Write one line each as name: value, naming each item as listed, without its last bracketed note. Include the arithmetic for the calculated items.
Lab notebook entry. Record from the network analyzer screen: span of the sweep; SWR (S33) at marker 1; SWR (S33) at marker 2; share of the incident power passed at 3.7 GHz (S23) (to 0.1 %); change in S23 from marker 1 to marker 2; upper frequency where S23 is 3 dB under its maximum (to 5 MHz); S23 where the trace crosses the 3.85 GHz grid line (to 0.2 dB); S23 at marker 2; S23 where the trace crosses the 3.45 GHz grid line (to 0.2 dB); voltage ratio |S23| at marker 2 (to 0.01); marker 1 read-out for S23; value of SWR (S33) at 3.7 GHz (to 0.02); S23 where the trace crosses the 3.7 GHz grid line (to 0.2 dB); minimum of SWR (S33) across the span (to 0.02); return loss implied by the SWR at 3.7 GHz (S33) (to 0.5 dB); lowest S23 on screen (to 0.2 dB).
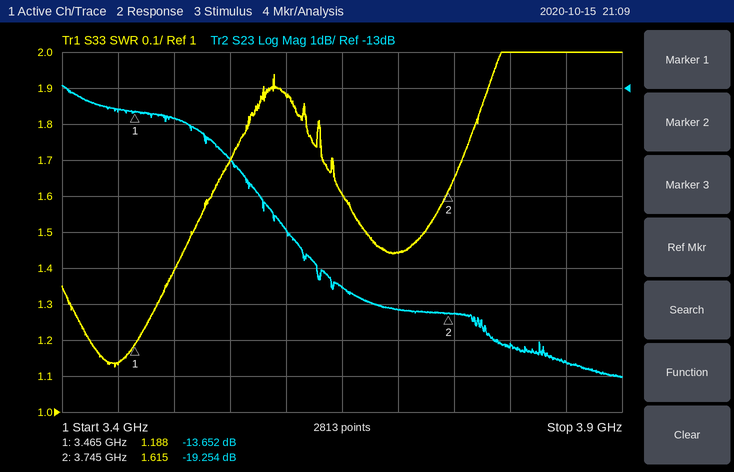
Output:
span of the sweep: 500 MHz
SWR (S33) at marker 1: 1.188
SWR (S33) at marker 2: 1.615
share of the incident power passed at 3.7 GHz (S23): 10^(-19.2/10) ≈ 1.2 %
change in S23 from marker 1 to marker 2: -19.254 − (-13.652) = -5.602 dB
upper frequency where S23 is 3 dB under its maximum: 3.575 GHz
S23 where the trace crosses the 3.85 GHz grid line: -20.6 dB
S23 at marker 2: -19.254 dB
S23 where the trace crosses the 3.45 GHz grid line: -13.6 dB
voltage ratio |S23| at marker 2: 10^(-19.254/20) ≈ 0.11
marker 1 read-out for S23: -13.652 dB
value of SWR (S33) at 3.7 GHz: 1.44
S23 where the trace crosses the 3.7 GHz grid line: -19.2 dB
minimum of SWR (S33) across the span: 1.12
return loss implied by the SWR at 3.7 GHz (S33): −20 log10((1.44 − 1)/(1.44 + 1)) ≈ 14.9 dB, so 15.0 dB to the nearest 0.5 dB
lowest S23 on screen: -21.0 dB
